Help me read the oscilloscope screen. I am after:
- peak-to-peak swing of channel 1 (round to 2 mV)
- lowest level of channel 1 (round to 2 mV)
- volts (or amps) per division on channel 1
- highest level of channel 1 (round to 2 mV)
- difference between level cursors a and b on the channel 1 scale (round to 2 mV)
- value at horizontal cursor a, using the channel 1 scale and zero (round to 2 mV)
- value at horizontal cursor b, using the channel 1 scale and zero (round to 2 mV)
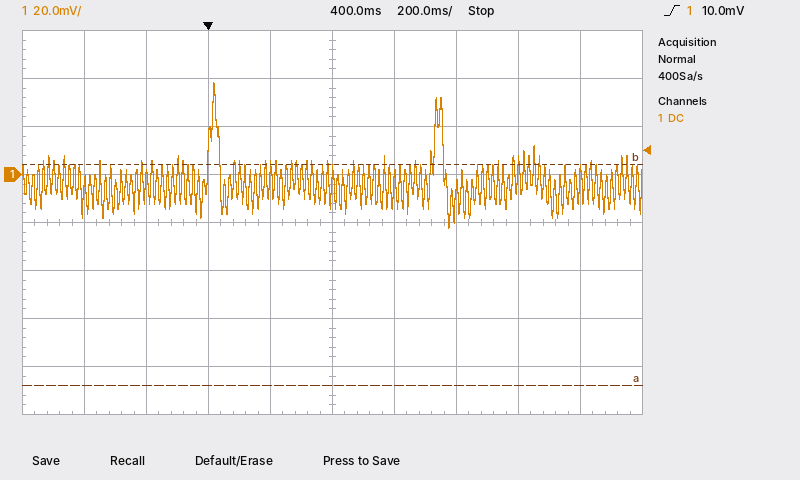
60 mV
-22 mV
20 mV
38 mV
92 mV
-88 mV
4 mV
